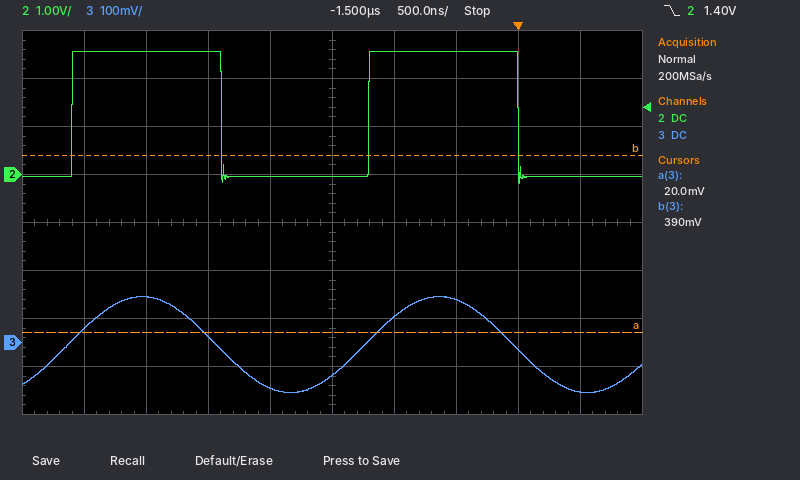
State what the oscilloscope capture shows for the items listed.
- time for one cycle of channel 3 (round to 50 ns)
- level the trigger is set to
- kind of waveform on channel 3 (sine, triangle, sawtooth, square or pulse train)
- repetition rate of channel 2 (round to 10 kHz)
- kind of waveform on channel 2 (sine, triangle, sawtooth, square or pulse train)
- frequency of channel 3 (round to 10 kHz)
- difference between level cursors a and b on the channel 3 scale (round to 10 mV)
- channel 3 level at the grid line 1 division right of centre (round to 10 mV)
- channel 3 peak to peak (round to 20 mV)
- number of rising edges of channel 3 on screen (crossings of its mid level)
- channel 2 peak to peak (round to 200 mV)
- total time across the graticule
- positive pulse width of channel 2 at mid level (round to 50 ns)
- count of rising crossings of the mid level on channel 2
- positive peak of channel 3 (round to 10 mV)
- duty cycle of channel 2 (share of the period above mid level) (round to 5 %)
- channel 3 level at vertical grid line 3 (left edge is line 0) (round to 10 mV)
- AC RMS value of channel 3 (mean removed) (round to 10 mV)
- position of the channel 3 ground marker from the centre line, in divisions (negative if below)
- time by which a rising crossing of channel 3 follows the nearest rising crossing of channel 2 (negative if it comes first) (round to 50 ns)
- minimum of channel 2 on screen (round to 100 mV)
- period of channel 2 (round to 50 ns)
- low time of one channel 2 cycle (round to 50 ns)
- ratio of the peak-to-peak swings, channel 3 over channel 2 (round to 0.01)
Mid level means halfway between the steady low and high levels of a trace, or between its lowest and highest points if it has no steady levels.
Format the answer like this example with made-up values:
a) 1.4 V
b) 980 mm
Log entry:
a) 2.40 µs
b) 1.40 V
c) sine
d) 420 kHz
e) square
f) 420 kHz
g) 370 mV
h) 50 mV
i) 200 mV
j) 2
k) 2.8 V
l) 5 µs
m) 1.20 µs
n) 2
o) 100 mV
p) 50 %
q) 10 mV
r) 70 mV
s) -2.5 div
t) -50 ns
u) -200 mV
v) 2.40 µs
w) 1.20 µs
x) 0.07
